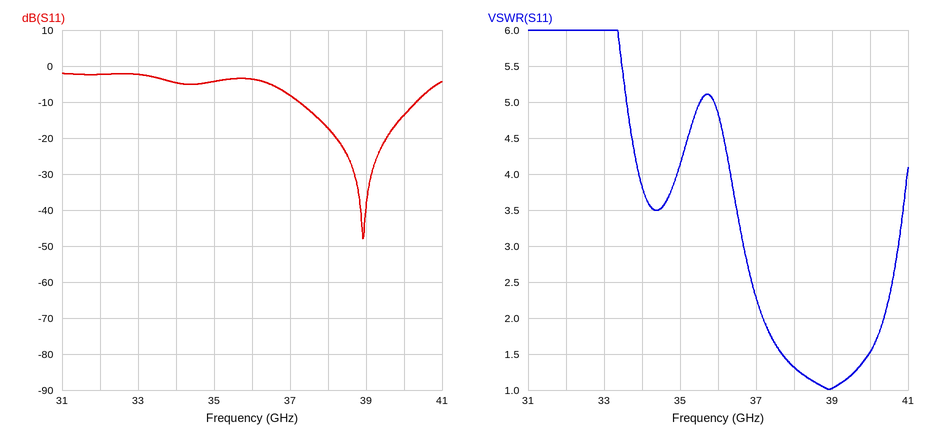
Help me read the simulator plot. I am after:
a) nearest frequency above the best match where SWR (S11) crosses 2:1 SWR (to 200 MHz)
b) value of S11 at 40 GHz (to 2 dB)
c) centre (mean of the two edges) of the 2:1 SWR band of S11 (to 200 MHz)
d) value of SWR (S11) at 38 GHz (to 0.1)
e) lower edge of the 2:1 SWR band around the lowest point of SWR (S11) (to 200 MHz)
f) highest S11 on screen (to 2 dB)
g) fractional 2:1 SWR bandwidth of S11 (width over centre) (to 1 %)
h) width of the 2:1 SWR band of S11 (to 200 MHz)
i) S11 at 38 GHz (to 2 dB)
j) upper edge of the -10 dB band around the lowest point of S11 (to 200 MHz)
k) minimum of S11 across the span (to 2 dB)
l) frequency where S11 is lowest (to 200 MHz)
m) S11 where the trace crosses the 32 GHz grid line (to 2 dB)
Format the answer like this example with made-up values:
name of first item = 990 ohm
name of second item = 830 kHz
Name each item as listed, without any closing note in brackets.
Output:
nearest frequency above the best match where SWR (S11) crosses 2:1 SWR = 40.4 GHz
value of S11 at 40 GHz = -14 dB
centre (mean of the two edges) of the 2:1 SWR band of S11 = 38.8 GHz
value of SWR (S11) at 38 GHz = 1.3
lower edge of the 2:1 SWR band around the lowest point of SWR (S11) = 37.2 GHz
highest S11 on screen = -2 dB
fractional 2:1 SWR bandwidth of S11 (width over centre) = 8 %
width of the 2:1 SWR band of S11 = 3.2 GHz
S11 at 38 GHz = -18 dB
upper edge of the -10 dB band around the lowest point of S11 = 40.4 GHz
minimum of S11 across the span = -48 dB
frequency where S11 is lowest = 39.0 GHz
S11 where the trace crosses the 32 GHz grid line = -2 dB
